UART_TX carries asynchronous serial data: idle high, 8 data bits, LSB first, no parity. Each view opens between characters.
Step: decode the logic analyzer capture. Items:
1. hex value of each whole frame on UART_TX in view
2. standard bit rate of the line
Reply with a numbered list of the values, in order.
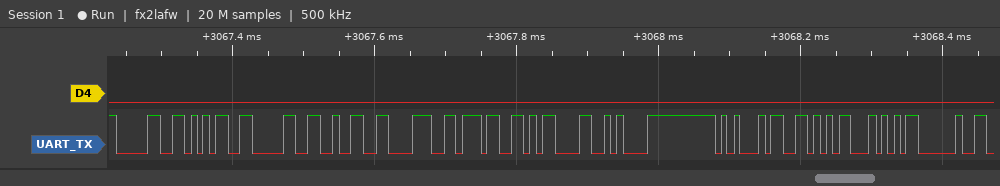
1. 30, 35, 30, 32, 38, 37, 0D, 0A, 45, 56, 54, 20
2. 115200 baud
